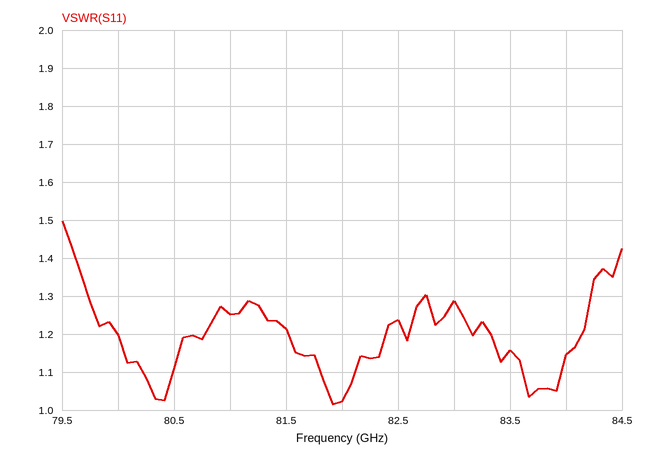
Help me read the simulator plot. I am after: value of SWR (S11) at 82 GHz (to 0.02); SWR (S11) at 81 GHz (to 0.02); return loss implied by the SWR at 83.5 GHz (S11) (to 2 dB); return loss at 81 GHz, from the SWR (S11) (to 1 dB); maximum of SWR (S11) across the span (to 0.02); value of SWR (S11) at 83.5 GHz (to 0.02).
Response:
1.02
1.26
22 dB
19 dB
1.50
1.16
